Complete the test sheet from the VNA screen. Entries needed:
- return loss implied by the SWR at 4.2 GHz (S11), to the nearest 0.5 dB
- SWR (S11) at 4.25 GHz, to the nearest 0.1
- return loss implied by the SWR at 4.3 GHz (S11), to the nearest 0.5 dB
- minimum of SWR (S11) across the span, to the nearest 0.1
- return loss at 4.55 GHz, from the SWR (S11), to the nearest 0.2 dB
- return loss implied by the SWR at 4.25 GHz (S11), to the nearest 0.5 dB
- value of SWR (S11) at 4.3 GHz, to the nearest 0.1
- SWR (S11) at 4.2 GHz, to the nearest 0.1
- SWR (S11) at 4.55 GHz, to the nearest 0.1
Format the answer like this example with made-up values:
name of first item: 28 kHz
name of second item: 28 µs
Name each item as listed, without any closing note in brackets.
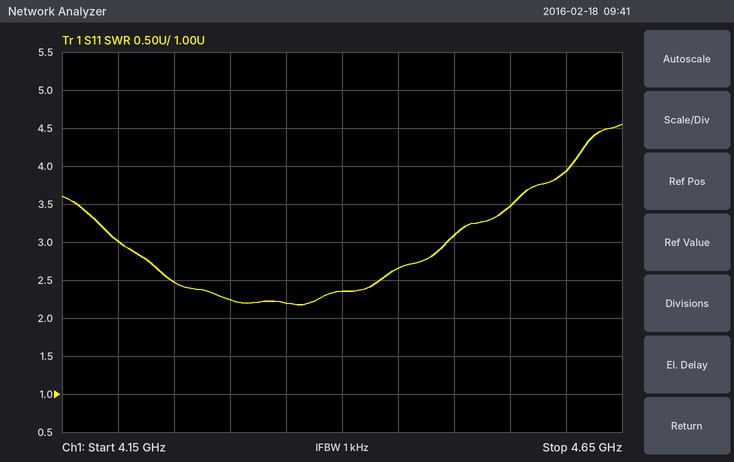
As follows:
return loss implied by the SWR at 4.2 GHz (S11), to the nearest 0.5 dB: 6.0 dB
SWR (S11) at 4.25 GHz, to the nearest 0.1: 2.5
return loss implied by the SWR at 4.3 GHz (S11), to the nearest 0.5 dB: 8.5 dB
minimum of SWR (S11) across the span, to the nearest 0.1: 2.2
return loss at 4.55 GHz, from the SWR (S11), to the nearest 0.2 dB: 5.2 dB
return loss implied by the SWR at 4.25 GHz (S11), to the nearest 0.5 dB: 7.5 dB
value of SWR (S11) at 4.3 GHz, to the nearest 0.1: 2.2
SWR (S11) at 4.2 GHz, to the nearest 0.1: 3.0
SWR (S11) at 4.55 GHz, to the nearest 0.1: 3.5
